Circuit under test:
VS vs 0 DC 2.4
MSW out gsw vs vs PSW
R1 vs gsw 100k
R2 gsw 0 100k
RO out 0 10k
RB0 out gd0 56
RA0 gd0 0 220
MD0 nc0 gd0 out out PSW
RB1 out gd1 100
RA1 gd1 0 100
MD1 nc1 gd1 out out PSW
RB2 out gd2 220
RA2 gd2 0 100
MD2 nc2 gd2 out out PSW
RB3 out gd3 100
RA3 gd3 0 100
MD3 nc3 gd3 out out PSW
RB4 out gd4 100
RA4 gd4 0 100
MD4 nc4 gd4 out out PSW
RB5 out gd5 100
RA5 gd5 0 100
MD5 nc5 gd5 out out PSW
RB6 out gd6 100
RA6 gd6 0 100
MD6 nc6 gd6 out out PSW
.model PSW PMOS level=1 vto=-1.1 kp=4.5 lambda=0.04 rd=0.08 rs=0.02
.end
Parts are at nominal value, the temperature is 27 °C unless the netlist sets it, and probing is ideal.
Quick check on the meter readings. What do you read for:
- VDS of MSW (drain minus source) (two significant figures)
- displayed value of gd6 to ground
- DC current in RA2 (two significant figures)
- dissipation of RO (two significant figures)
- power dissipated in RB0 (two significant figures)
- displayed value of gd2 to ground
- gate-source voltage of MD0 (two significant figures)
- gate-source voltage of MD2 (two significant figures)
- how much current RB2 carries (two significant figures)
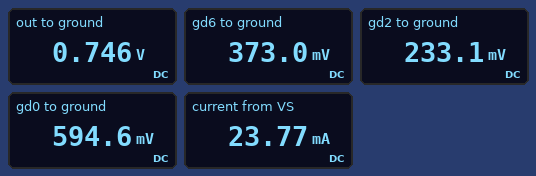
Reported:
-1.7 V
373.0 mV
2.3 mA
56 µW
410 µW
233.1 mV
-150 mV
-510 mV
2.3 mA
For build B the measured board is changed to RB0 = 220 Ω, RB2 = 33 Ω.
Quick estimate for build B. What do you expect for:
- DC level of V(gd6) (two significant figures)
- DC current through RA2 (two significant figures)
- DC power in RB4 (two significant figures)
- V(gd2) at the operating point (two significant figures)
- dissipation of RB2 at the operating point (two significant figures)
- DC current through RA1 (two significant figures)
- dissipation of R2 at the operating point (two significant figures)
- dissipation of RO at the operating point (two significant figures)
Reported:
340 mV
5.1 mA
1.2 mW
510 mV
870 µW
3.4 mA
14 µW
47 µW
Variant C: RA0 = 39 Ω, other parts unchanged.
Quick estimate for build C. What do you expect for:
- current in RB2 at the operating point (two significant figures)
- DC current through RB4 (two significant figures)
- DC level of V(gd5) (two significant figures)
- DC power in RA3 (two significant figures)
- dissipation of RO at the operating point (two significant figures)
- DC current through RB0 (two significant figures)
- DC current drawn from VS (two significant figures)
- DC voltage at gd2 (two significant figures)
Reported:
1.9 mA
3.1 mA
310 mV
950 µW
38 µW
6.5 mA
24 mA
190 mV
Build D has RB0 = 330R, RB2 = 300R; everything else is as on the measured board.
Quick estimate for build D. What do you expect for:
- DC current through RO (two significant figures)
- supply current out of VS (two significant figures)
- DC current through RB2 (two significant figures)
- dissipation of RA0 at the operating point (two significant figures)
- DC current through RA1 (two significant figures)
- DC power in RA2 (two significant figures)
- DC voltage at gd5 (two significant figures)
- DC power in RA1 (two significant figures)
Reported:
81 µA
24 mA
2.0 mA
470 µW
4.0 mA
410 µW
400 mV
1.6 mW
